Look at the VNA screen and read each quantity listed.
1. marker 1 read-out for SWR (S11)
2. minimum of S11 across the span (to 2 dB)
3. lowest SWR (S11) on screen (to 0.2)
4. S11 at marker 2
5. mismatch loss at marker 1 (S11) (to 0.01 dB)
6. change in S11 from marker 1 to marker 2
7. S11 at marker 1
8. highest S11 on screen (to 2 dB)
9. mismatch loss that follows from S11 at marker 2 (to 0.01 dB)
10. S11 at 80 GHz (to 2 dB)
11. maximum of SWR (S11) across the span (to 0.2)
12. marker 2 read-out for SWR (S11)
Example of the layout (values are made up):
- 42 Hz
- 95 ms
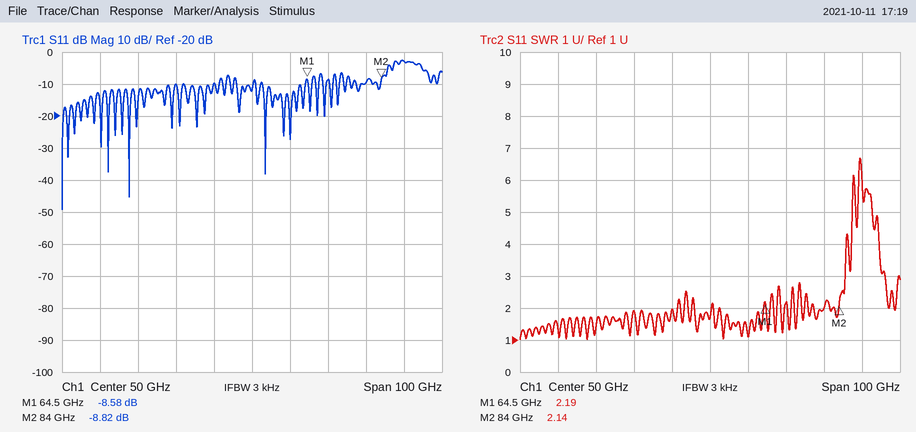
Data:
- 2.19
- -50 dB
- 1.0
- -8.82 dB
- 0.65 dB
- -0.24 dB
- -8.58 dB
- -2 dB
- 0.61 dB
- -10 dB
- 6.6
- 2.14
